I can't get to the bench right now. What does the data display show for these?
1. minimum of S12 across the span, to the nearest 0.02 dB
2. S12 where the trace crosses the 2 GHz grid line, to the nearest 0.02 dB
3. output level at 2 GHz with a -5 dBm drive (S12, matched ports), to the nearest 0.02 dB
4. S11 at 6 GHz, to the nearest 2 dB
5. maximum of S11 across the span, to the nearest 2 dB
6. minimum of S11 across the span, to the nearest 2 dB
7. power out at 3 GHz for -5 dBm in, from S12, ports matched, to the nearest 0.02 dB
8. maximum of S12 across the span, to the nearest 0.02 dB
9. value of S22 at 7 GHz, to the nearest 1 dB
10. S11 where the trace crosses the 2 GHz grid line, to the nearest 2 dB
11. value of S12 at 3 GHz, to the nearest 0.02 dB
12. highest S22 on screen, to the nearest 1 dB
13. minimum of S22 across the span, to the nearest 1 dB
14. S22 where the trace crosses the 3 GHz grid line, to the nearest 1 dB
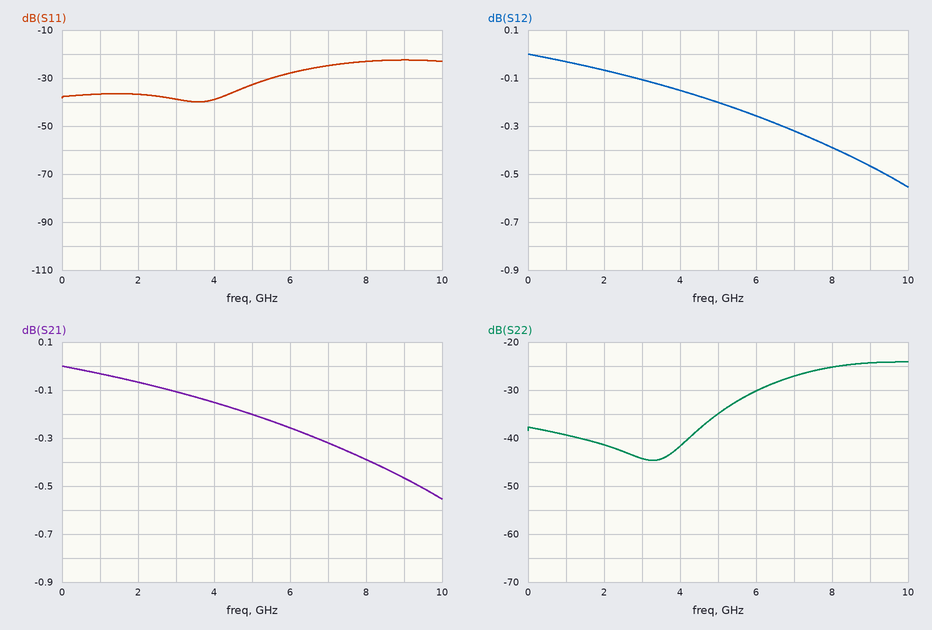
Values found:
-0.56 dB
-0.06 dB
-5.06 dBm
-28 dB
-22 dB
-40 dB
-5.10 dBm
0.00 dB
-27 dB
-36 dB
-0.10 dB
-24 dB
-45 dB
-44 dB
